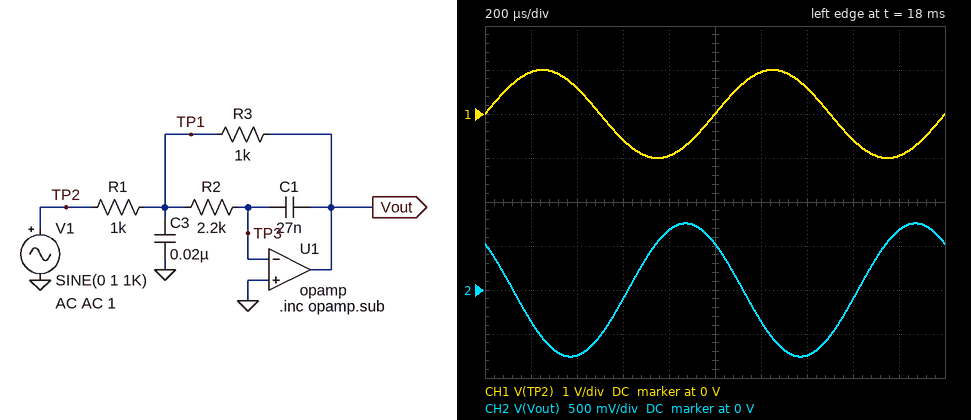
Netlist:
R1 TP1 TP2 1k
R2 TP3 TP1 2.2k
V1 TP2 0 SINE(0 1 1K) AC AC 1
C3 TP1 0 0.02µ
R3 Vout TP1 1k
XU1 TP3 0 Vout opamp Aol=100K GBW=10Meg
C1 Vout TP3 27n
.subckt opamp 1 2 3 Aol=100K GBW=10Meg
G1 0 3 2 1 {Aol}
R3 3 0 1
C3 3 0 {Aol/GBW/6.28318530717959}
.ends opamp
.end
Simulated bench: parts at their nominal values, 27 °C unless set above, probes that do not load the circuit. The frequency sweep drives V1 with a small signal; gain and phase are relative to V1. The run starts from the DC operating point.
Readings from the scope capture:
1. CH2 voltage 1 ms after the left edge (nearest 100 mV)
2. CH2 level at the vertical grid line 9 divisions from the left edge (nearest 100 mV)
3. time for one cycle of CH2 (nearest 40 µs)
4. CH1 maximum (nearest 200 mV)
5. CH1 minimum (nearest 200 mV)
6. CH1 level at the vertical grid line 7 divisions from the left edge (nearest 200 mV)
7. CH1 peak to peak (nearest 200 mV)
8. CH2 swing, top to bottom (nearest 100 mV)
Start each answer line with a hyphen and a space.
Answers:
- 500 mV
- 700 mV
- 1.00 ms
- 1.0 V
- -1.0 V
- 600 mV
- 2.0 V
- 1.5 V
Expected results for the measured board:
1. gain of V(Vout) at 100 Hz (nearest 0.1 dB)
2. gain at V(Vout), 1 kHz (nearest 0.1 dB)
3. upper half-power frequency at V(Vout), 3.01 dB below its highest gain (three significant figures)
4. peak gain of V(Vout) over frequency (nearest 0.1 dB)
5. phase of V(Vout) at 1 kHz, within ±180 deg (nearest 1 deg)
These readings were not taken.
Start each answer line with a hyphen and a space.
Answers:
- 0 dB
- -2.4 dB
- 1.16 kHz
- 0 dB
- 136 deg
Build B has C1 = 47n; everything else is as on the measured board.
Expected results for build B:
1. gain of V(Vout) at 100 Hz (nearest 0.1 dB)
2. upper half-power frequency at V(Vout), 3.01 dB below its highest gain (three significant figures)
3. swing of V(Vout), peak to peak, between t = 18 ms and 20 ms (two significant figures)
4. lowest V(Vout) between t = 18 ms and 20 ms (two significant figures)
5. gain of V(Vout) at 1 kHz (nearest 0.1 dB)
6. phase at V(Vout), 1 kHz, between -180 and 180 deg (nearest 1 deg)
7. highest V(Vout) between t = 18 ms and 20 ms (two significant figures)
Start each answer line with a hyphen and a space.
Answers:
- -0.1 dB
- 648 Hz
- 1.1 V
- -540 mV
- -5.3 dB
- 120 deg
- 540 mV
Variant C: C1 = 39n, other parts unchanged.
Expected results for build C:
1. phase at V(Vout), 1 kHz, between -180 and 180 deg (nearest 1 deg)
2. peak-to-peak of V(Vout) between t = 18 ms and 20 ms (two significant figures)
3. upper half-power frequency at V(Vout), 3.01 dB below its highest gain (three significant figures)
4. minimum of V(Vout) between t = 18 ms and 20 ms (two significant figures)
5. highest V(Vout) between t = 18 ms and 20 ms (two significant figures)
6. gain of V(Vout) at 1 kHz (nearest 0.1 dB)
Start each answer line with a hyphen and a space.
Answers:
- 125 deg
- 1.2 V
- 786 Hz
- -620 mV
- 620 mV
- -4.2 dB
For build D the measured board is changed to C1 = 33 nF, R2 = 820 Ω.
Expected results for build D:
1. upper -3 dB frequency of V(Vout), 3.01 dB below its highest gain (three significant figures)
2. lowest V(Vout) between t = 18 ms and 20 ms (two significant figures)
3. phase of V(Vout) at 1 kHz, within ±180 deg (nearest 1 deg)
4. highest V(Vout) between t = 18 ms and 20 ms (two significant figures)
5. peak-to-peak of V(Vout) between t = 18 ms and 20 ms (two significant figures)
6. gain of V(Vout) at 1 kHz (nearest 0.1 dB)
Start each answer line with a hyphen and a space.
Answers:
- 1.97 kHz
- -890 mV
- 151 deg
- 890 mV
- 1.8 V
- -1.0 dB
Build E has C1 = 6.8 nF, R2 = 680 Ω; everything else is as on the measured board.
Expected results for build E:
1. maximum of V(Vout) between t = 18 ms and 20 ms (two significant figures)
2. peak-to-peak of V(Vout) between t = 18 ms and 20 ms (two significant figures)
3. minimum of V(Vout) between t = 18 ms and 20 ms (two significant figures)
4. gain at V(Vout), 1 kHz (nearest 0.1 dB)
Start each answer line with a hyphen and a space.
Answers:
- 1.0 V
- 2.0 V
- -1.0 V
- 0 dB
